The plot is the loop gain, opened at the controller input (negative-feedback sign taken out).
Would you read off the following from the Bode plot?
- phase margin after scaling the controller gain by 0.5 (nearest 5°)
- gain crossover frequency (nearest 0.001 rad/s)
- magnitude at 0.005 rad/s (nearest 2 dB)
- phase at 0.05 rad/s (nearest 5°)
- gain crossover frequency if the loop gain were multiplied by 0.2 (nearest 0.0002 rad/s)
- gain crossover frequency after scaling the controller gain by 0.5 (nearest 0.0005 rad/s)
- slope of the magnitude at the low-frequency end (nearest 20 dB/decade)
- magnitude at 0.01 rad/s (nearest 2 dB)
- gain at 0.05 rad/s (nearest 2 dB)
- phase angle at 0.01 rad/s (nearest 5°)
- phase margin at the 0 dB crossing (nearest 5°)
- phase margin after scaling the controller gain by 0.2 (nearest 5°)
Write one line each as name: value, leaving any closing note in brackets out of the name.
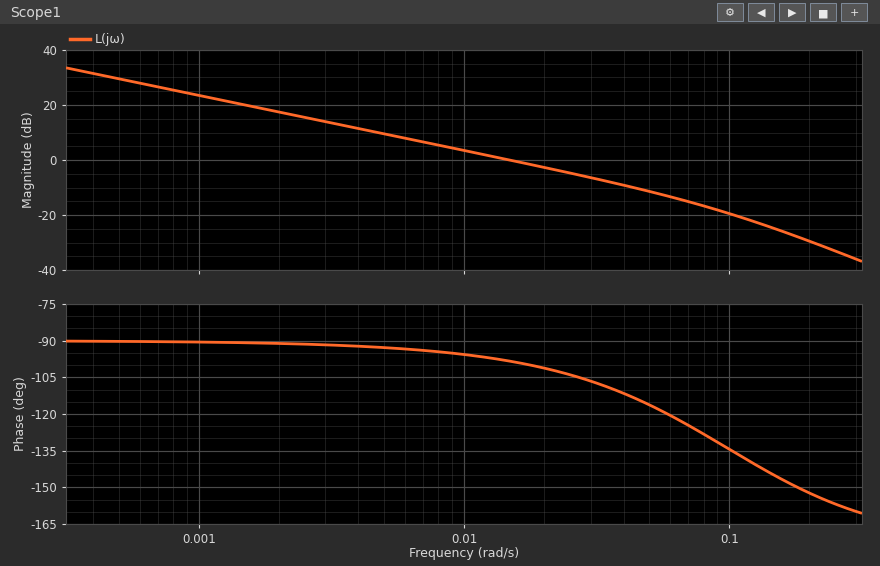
phase margin after scaling the controller gain by 0.5: 85°
gain crossover frequency: 0.015 rad/s
magnitude at 0.005 rad/s: 10 dB
phase at 0.05 rad/s: -115°
gain crossover frequency if the loop gain were multiplied by 0.2: 0.0030 rad/s
gain crossover frequency after scaling the controller gain by 0.5: 0.0075 rad/s
slope of the magnitude at the low-frequency end: -20 dB/decade
magnitude at 0.01 rad/s: 4 dB
gain at 0.05 rad/s: -12 dB
phase angle at 0.01 rad/s: -95°
phase margin at the 0 dB crossing: 80°
phase margin after scaling the controller gain by 0.2: 90°
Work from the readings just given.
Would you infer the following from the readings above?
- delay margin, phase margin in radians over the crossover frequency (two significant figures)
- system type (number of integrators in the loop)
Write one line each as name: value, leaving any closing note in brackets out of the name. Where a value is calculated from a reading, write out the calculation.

delay margin, phase margin in radians over the crossover frequency: 80 × π / 180 / 0.015 = 93 s
system type: 1
